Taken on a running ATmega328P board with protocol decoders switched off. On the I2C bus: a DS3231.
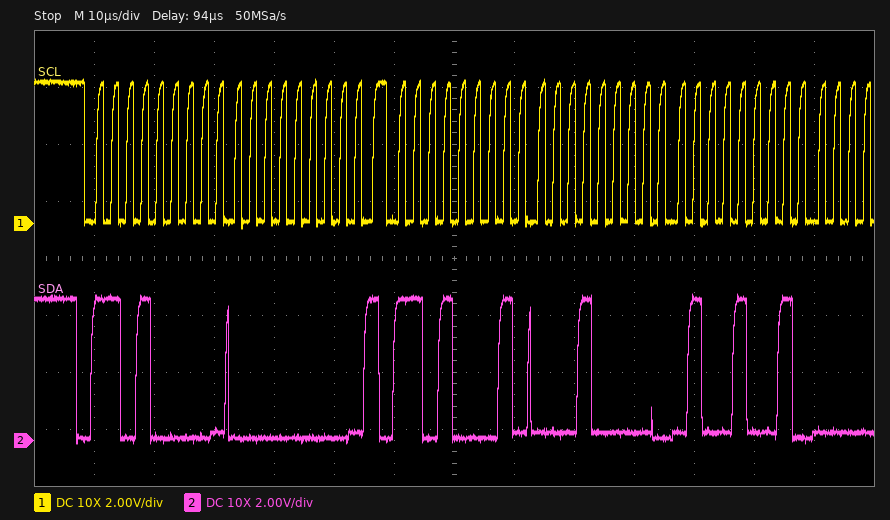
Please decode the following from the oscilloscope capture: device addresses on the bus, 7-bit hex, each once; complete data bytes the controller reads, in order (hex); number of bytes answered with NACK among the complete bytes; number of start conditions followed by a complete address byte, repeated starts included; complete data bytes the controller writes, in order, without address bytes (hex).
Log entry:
0x68
10 49
0
2
00
